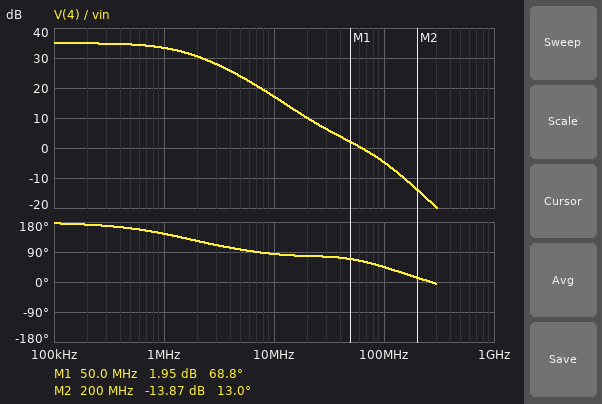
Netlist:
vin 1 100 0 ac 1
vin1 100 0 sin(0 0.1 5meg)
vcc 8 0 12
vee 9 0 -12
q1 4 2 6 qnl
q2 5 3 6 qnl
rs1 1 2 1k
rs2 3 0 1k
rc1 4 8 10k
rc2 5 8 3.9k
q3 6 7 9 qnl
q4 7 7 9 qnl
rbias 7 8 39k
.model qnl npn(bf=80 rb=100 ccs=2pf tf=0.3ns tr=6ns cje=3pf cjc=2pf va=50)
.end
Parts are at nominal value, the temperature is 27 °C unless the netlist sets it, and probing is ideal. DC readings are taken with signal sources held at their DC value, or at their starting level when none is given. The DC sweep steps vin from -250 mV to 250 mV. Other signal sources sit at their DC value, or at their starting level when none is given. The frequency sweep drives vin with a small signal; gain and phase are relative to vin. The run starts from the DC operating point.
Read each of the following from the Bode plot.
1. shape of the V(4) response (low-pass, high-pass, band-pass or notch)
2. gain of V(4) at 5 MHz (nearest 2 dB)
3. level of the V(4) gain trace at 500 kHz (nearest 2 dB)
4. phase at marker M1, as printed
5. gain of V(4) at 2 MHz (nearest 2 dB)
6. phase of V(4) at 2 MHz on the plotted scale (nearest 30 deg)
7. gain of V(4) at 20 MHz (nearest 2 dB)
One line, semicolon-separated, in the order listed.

low-pass; 24 dB; 34 dB; 68.8 deg; 30 dB; 120 deg; 10 dB
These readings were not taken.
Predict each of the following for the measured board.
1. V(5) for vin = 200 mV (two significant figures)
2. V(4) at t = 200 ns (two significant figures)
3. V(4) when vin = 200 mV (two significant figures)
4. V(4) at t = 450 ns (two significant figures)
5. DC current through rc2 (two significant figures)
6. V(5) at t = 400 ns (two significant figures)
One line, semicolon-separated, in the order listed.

12 V; 9.9 V; 5.0 V; 8.3 V; 350 µA; 10 V
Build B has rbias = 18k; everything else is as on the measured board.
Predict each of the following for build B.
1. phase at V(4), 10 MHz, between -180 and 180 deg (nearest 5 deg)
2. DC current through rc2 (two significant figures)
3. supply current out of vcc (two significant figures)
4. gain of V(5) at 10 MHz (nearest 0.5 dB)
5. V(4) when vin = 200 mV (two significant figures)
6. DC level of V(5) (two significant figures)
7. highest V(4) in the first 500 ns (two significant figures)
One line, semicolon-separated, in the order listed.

80 deg; 780 µA; 2.8 mA; 14.5 dB; -650 mV; 9.0 V; 6.2 V
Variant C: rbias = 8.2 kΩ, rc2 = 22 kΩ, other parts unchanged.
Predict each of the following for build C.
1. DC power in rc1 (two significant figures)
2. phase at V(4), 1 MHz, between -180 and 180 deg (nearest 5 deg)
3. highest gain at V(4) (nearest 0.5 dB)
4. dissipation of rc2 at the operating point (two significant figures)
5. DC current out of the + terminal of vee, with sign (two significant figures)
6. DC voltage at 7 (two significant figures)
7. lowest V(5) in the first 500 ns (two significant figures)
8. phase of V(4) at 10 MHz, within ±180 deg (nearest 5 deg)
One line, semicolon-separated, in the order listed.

18 mW; -5 deg; -7.0 dB; 8.3 mW; -6.1 mA; -11 V; -1.5 V; -25 deg
